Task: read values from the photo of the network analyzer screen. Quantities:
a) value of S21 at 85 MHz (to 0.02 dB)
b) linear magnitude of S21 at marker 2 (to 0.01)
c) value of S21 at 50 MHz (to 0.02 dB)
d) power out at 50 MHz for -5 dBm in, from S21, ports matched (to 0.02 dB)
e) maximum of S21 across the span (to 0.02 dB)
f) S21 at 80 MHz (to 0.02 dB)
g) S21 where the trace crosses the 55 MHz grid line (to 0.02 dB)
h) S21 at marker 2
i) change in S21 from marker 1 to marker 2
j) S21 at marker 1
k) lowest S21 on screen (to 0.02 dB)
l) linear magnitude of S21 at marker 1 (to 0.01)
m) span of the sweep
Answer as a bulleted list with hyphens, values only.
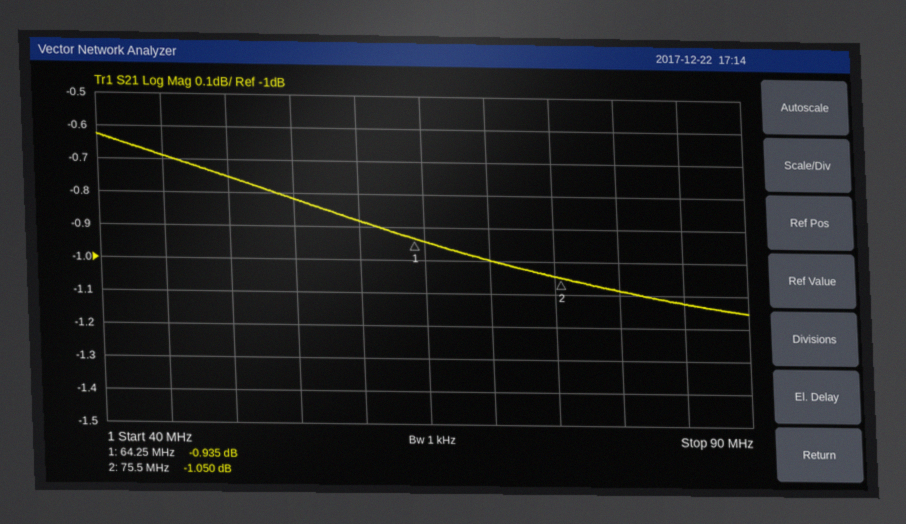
- -1.12 dB
- 0.89
- -0.76 dB
- -5.76 dBm
- -0.62 dB
- -1.08 dB
- -0.82 dB
- -1.050 dB
- -0.115 dB
- -0.935 dB
- -1.16 dB
- 0.90
- 50 MHz
